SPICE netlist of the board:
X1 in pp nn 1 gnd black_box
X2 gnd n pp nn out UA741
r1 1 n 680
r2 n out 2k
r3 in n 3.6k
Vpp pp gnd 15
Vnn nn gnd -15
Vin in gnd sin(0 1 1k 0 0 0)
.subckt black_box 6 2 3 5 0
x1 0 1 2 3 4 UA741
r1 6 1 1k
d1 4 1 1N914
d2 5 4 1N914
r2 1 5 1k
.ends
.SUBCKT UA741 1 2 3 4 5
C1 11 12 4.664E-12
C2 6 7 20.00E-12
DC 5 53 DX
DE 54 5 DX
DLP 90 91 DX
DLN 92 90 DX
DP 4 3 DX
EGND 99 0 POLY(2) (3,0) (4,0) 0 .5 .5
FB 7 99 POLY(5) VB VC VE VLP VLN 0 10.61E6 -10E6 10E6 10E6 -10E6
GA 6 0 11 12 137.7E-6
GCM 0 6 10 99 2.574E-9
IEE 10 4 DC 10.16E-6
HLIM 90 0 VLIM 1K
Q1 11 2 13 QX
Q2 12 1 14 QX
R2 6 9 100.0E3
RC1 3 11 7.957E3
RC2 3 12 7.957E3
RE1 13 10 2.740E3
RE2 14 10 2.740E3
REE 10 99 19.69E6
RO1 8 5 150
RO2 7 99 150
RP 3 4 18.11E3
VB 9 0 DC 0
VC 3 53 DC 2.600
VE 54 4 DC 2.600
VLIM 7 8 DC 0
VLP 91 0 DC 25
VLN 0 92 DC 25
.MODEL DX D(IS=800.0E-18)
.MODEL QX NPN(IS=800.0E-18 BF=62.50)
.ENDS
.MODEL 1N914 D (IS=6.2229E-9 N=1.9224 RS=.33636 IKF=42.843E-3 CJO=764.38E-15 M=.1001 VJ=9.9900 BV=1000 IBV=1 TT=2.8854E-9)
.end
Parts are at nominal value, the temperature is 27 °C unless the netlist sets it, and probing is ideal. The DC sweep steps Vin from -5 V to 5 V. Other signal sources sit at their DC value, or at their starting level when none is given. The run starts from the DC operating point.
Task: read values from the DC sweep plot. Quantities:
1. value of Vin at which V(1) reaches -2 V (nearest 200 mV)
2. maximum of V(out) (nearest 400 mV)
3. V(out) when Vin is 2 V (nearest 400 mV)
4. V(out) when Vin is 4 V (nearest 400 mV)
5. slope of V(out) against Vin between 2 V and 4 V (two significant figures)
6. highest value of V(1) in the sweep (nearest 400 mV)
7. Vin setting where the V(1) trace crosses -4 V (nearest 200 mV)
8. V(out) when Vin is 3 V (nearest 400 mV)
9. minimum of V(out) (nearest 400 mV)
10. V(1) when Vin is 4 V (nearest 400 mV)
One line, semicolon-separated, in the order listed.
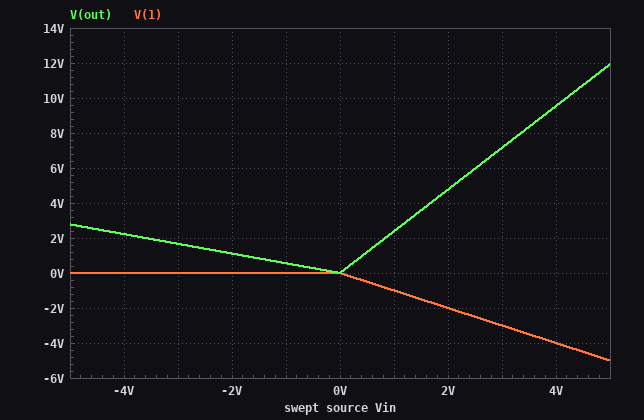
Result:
2.0 V; 12.0 V; 4.8 V; 9.6 V; 2.4 V/V; 0 V; 4.0 V; 7.2 V; 0 V; -4.0 V
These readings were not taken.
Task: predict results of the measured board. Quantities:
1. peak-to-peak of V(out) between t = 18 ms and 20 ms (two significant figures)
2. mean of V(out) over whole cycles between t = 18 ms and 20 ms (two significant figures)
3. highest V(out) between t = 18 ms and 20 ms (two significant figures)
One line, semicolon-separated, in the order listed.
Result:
2.4 V; 940 mV; 2.4 V
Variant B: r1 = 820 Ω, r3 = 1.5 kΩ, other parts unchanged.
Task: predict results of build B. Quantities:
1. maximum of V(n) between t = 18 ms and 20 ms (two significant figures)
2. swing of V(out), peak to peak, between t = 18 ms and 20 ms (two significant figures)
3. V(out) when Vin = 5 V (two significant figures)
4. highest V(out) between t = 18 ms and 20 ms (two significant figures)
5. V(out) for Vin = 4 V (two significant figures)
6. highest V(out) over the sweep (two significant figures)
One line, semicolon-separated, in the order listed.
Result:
2.0 mV; 1.4 V; 5.5 V; 1.3 V; 4.4 V; 6.7 V
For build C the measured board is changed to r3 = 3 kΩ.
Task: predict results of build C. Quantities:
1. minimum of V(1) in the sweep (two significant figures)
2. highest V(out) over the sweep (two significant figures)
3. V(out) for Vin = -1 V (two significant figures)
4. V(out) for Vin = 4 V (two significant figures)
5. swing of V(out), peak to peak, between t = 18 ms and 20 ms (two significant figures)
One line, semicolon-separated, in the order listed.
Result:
-5.0 V; 11 V; 670 mV; 9.1 V; 2.3 V
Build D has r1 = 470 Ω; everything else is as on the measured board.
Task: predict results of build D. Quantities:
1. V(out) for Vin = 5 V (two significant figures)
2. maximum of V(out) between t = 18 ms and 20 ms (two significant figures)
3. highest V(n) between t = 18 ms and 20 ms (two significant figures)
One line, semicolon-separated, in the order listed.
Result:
13 V; 3.7 V; 3.6 mV
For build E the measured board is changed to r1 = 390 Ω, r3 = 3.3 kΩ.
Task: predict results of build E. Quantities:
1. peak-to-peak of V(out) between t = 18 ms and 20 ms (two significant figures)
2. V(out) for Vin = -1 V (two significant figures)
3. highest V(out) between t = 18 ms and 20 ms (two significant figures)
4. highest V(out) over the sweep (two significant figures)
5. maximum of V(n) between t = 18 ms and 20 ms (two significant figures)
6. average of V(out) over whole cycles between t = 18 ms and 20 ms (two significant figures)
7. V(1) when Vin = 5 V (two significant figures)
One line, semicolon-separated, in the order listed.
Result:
4.6 V; 610 mV; 4.5 V; 13 V; 4.4 mV; 1.6 V; -5.0 V
